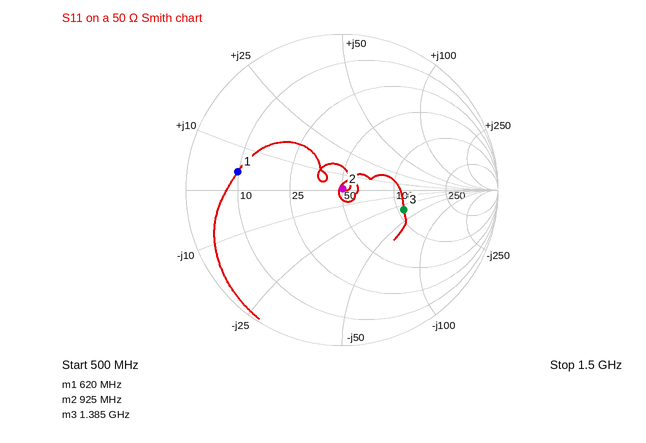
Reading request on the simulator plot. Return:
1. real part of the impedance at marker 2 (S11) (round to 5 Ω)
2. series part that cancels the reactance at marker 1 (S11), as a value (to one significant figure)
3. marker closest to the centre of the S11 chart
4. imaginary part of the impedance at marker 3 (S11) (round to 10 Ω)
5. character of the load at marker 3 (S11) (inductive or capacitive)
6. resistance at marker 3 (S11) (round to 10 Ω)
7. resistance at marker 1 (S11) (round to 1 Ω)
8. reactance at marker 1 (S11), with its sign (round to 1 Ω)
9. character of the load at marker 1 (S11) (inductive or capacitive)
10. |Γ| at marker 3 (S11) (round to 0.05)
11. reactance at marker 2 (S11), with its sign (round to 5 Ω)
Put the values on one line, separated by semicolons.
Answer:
50 Ω; 60 pF; marker 2; -30 Ω; capacitive; 110 Ω; 10 Ω; +4 Ω; inductive; 0.40; 0 Ω
